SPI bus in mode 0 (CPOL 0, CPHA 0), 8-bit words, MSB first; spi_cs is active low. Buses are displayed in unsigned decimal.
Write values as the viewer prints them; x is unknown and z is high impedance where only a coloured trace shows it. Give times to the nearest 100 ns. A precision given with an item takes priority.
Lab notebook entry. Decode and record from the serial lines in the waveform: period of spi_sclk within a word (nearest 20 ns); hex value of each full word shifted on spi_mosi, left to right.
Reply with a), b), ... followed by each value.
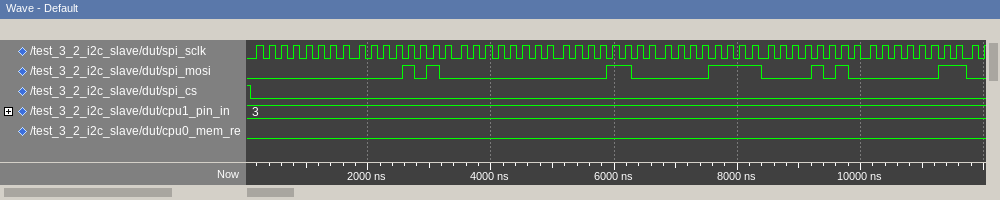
a) 200 ns
b) 00, 0A, 00, 0C, 0F, 0A, 03
